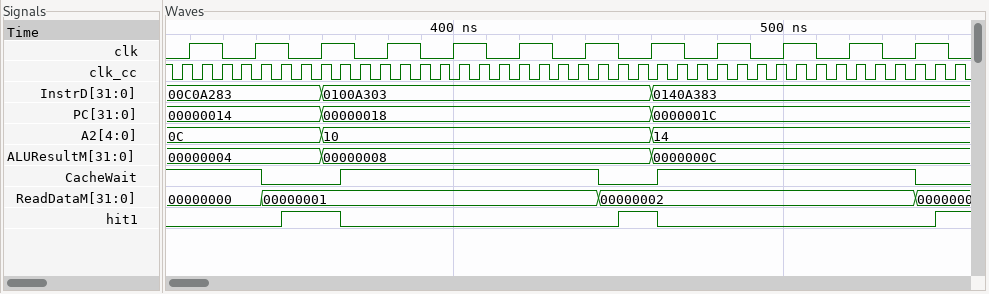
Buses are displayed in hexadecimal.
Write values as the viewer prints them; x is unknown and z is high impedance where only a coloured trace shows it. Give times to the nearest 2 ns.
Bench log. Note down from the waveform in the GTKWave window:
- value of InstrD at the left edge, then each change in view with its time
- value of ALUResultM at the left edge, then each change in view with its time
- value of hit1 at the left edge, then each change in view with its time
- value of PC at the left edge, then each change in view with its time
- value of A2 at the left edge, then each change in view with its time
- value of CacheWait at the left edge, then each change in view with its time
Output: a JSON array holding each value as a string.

["00C0A283, 0100A303 at 360 ns, 0140A383 at 460 ns", "00000004, 00000008 at 360 ns, 0000000C at 460 ns", "0, 1 at 348 ns, 0 at 366 ns, 1 at 450 ns, 0 at 462 ns, 1 at 546 ns", "00000014, 00000018 at 360 ns, 0000001C at 460 ns", "0C, 10 at 360 ns, 14 at 460 ns", "1, 0 at 342 ns, 1 at 366 ns, 0 at 444 ns, 1 at 462 ns, 0 at 540 ns"]
